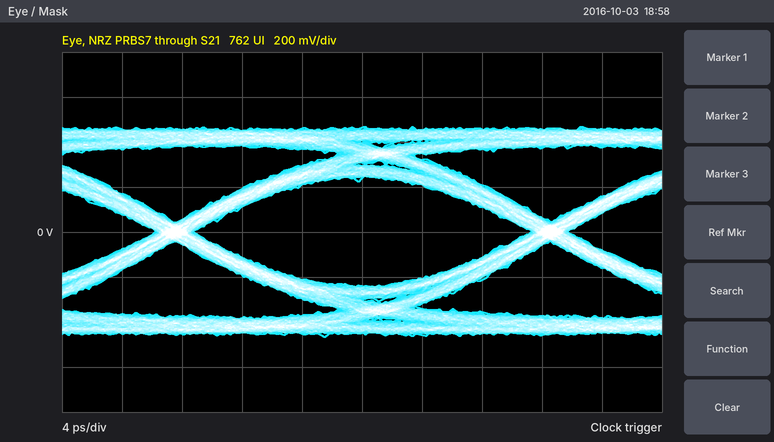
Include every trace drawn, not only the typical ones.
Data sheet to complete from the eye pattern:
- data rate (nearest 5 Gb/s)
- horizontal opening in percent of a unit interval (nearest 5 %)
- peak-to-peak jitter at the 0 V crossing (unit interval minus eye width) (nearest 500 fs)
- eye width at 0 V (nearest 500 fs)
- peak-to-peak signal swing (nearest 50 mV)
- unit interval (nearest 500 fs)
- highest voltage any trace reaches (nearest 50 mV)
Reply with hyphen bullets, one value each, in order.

- 40 Gb/s
- 90 %
- 2.5 ps
- 22.5 ps
- 950 mV
- 25.0 ps
- 450 mV
